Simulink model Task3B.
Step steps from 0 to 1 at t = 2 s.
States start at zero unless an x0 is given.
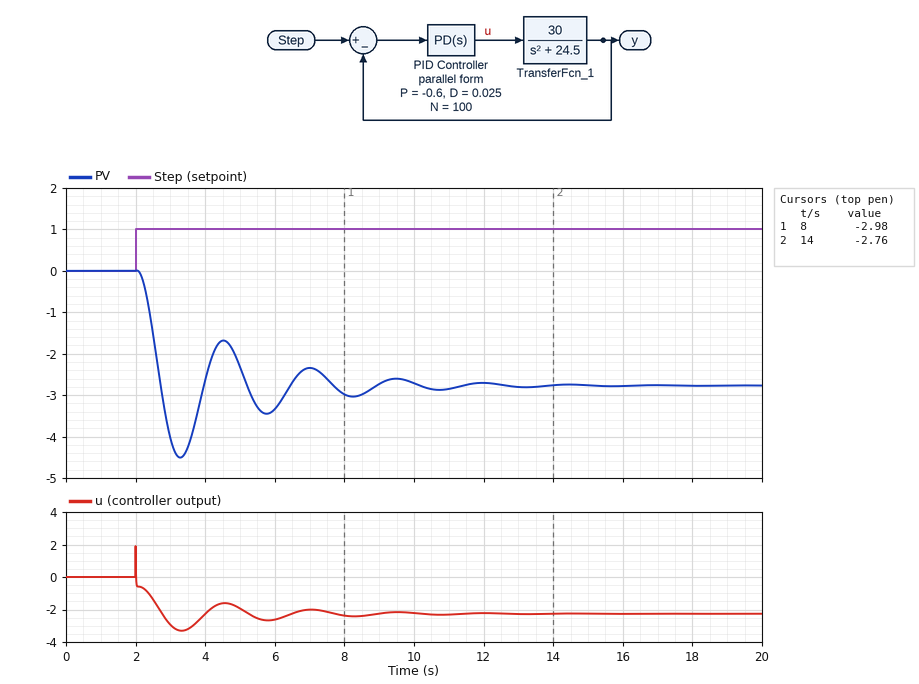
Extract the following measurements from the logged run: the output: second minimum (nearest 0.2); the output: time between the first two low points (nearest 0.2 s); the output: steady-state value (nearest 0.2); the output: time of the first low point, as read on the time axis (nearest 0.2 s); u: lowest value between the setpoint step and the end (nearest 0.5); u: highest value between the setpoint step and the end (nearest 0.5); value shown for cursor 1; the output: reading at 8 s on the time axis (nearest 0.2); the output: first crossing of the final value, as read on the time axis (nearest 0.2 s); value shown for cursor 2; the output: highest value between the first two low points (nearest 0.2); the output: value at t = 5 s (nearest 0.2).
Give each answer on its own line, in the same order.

-3.4
2.4 s
-2.8
3.2 s
-3.5
2.0
-2.98
-3.0
2.8 s
-2.76
-1.6
-2.4
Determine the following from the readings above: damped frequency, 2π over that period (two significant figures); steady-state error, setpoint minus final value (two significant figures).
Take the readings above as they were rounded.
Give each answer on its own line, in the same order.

2.6 rad/s
3.8
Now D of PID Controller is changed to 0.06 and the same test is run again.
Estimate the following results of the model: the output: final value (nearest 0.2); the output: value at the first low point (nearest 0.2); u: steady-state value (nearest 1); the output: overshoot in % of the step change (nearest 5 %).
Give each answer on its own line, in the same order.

-2.8
-3.6
-2
30 %
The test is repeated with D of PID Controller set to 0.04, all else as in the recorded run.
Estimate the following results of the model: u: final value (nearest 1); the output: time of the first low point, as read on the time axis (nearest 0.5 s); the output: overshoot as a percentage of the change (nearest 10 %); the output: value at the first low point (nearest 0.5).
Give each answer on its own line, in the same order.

-2
3.5 s
50 %
-4.0
